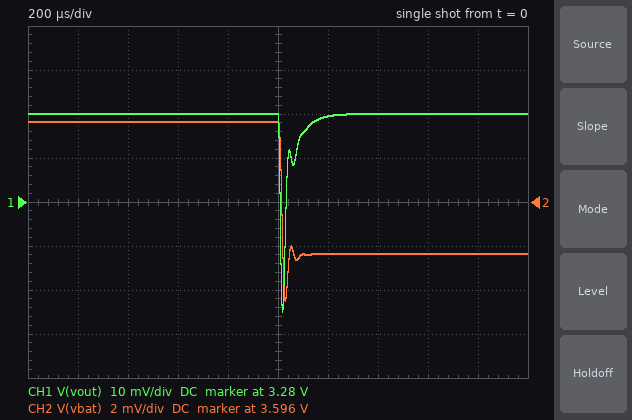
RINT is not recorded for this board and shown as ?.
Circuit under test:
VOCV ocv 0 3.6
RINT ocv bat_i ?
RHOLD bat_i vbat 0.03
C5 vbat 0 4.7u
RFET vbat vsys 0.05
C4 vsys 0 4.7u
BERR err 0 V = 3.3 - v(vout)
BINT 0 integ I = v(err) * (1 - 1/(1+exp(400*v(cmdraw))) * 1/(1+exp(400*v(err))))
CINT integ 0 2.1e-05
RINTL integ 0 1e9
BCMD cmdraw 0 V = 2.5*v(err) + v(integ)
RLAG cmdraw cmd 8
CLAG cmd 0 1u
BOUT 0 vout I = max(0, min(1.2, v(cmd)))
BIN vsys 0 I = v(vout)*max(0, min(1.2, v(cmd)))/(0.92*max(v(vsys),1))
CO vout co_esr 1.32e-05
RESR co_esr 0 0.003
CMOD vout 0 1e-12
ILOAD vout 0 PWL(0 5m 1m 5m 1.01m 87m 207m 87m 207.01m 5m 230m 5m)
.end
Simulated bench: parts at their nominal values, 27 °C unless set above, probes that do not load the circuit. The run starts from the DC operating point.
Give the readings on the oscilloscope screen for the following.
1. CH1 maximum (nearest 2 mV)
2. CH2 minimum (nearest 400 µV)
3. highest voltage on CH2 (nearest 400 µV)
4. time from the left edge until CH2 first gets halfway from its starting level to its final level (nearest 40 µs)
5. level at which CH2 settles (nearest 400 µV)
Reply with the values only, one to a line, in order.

3.300 V
3.5916 V
3.5996 V
1.00 ms
3.5936 V
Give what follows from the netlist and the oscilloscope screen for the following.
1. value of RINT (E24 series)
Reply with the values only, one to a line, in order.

0.043 Ω
